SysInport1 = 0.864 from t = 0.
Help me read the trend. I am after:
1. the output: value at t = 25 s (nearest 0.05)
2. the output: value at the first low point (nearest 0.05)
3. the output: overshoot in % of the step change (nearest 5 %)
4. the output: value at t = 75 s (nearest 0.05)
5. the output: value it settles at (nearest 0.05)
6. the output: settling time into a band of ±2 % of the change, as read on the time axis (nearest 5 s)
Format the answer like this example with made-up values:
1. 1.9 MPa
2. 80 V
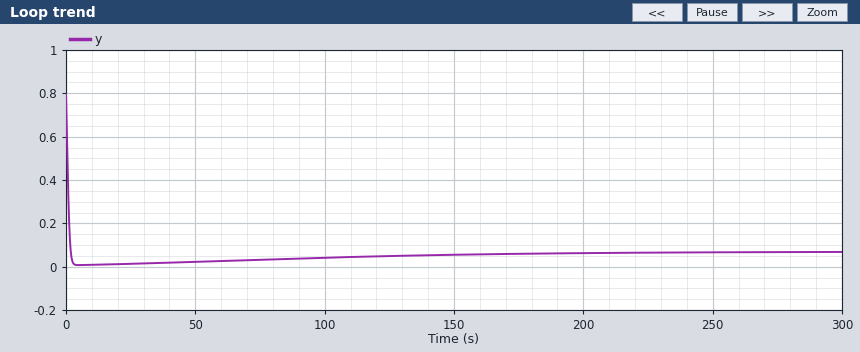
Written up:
1. 0.00
2. 0.00
3. 10 %
4. 0.05
5. 0.05
6. 150 s
